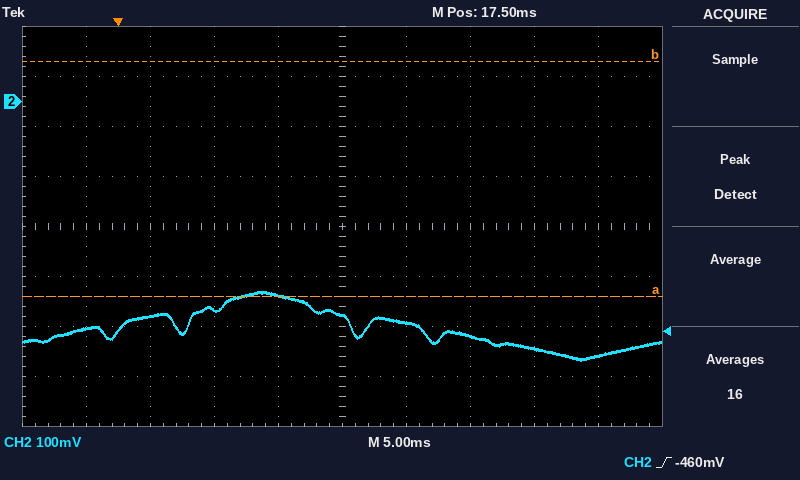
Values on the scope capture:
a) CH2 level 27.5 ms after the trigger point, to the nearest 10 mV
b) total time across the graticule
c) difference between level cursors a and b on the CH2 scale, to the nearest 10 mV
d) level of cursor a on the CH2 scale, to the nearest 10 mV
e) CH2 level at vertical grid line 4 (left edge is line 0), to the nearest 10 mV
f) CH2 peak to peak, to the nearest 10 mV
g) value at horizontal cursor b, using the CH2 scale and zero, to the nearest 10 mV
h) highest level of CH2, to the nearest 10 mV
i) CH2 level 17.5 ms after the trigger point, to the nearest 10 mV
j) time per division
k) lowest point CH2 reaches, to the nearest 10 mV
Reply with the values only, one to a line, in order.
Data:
-470 mV
50 ms
470 mV
-390 mV
-390 mV
140 mV
80 mV
-380 mV
-430 mV
5 ms
-520 mV
